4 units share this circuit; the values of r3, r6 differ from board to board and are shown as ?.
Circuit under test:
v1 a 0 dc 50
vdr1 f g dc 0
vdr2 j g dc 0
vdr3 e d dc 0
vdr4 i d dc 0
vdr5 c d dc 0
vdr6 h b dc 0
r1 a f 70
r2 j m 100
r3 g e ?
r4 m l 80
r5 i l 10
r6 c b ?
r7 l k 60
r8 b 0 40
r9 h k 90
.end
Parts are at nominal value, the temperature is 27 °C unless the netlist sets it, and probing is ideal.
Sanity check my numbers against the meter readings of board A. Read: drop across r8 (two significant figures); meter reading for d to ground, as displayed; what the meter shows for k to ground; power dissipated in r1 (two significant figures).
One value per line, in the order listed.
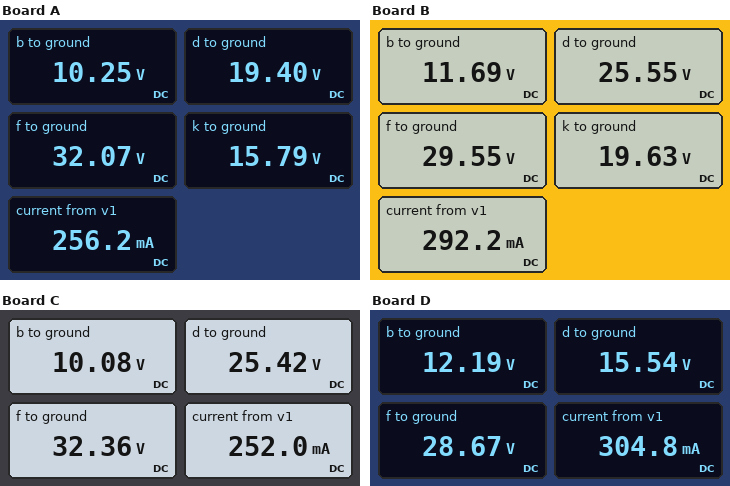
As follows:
10 V
19.40 V
15.79 V
4.6 W
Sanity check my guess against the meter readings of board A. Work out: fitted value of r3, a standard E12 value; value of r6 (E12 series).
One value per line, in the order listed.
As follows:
68 Ω
47 Ω
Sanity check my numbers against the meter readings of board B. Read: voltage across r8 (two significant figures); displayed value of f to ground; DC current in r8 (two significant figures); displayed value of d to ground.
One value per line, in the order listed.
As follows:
12 V
29.55 V
290 mA
25.55 V
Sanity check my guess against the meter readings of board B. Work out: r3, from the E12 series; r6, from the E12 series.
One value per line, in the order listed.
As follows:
15 Ω
68 Ω
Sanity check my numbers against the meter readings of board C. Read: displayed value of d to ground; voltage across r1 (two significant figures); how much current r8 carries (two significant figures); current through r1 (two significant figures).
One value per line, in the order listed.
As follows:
25.42 V
18 V
250 mA
250 mA
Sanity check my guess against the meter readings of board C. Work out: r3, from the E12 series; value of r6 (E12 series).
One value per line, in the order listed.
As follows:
33 Ω
100 Ω
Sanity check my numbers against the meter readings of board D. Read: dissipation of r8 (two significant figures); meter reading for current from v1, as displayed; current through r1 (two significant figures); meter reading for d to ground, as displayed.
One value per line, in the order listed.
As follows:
3.7 W
304.8 mA
300 mA
15.54 V
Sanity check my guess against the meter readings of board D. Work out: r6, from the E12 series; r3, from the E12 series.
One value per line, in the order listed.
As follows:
12 Ω
56 Ω
